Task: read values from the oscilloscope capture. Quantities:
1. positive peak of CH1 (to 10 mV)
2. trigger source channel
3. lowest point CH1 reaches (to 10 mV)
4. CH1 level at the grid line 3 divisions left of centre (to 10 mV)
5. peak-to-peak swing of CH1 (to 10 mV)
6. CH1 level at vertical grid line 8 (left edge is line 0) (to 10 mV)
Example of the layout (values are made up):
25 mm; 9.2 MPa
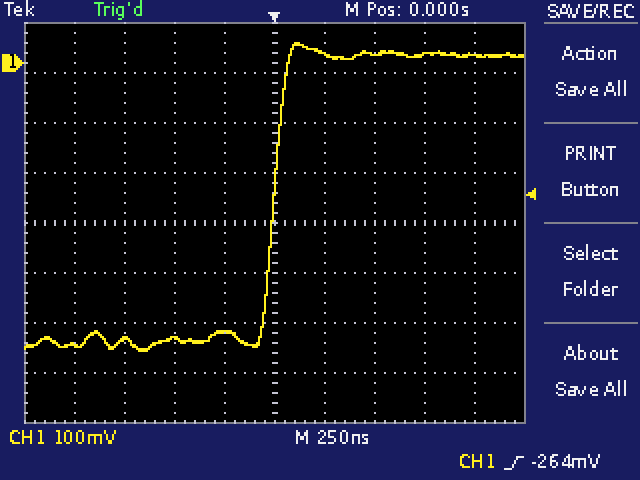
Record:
40 mV; CH1; -580 mV; -550 mV; 620 mV; 20 mV
